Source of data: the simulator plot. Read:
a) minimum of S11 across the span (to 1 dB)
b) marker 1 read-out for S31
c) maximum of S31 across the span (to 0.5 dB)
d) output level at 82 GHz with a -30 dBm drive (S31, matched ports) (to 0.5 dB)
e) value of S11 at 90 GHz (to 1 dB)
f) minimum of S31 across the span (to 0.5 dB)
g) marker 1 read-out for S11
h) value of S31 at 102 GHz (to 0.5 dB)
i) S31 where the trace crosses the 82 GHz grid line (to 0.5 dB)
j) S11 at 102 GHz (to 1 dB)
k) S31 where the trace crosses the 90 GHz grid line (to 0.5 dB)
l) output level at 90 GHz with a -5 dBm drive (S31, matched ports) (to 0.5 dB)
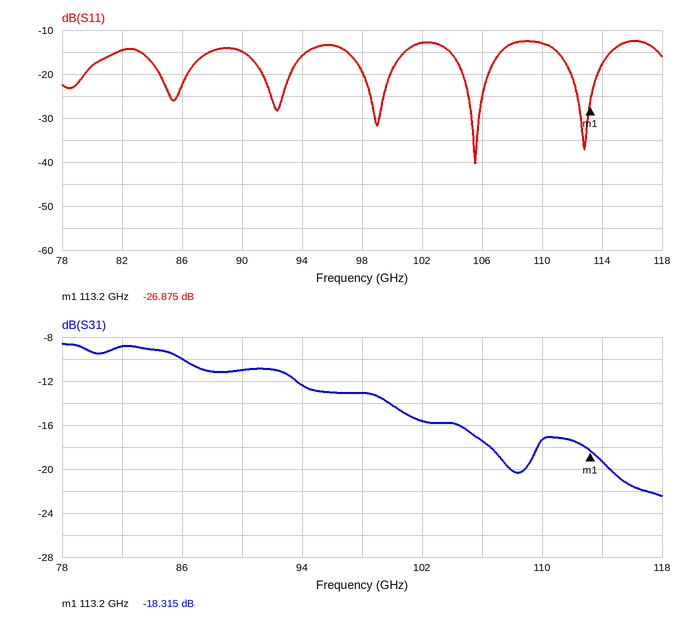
-40 dB
-18.315 dB
-8.5 dB
-39.0 dBm
-15 dB
-22.5 dB
-26.875 dB
-15.5 dB
-9.0 dB
-13 dB
-11.0 dB
-16.0 dBm
